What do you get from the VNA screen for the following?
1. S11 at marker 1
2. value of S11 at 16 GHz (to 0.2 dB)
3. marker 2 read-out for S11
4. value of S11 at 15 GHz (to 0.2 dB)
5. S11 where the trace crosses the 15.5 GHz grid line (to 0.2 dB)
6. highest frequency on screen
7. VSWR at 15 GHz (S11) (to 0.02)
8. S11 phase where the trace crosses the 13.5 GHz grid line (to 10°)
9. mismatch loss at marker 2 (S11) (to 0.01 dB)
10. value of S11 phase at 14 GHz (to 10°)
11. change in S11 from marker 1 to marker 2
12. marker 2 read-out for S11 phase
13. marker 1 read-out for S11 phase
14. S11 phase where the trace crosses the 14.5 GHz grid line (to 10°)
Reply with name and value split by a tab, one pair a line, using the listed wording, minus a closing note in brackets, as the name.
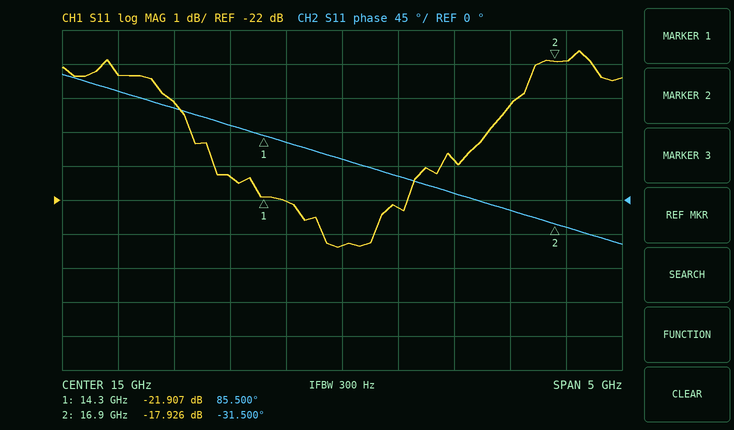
S11 at marker 1	-21.907 dB
value of S11 at 16 GHz	-20.8 dB
marker 2 read-out for S11	-17.926 dB
value of S11 at 15 GHz	-23.4 dB
S11 where the trace crosses the 15.5 GHz grid line	-22.2 dB
highest frequency on screen	17.5 GHz
VSWR at 15 GHz (S11)	1.14
S11 phase where the trace crosses the 13.5 GHz grid line	120°
mismatch loss at marker 2 (S11)	0.07 dB
value of S11 phase at 14 GHz	100°
change in S11 from marker 1 to marker 2	3.981 dB
marker 2 read-out for S11 phase	-31.500°
marker 1 read-out for S11 phase	85.500°
S11 phase where the trace crosses the 14.5 GHz grid line	80°
